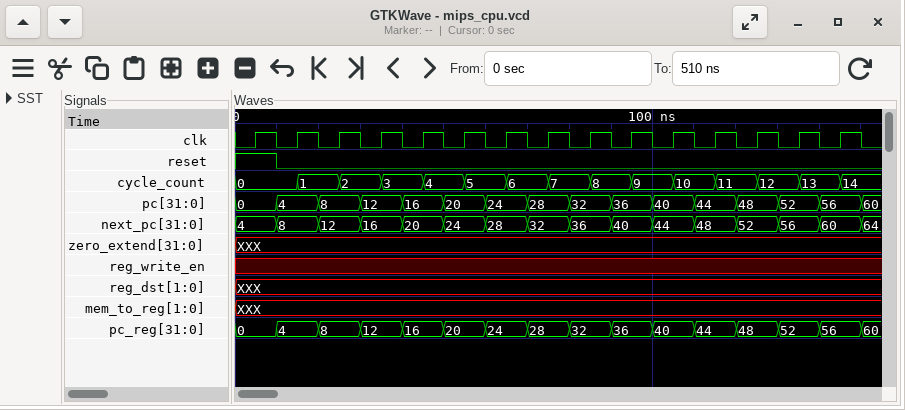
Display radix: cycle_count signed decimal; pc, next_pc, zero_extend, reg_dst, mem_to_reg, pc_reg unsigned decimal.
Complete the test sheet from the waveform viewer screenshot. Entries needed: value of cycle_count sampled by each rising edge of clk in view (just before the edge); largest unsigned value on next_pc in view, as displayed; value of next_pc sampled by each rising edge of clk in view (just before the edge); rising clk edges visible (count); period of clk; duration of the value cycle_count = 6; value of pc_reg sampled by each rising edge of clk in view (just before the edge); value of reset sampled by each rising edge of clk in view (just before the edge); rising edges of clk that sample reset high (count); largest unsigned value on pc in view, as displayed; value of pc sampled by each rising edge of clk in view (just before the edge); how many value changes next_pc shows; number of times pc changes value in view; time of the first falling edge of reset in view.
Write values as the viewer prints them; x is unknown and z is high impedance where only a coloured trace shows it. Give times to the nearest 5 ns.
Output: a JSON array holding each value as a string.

["0, 0, 1, 2, 3, 4, 5, 6, 7, 8, 9, 10, 11, 12, 13", "64", "4, 8, 12, 16, 20, 24, 28, 32, 36, 40, 44, 48, 52, 56, 60", "15", "10 ns", "10 ns", "0, 4, 8, 12, 16, 20, 24, 28, 32, 36, 40, 44, 48, 52, 56", "1 0 0 0 0 0 0 0 0 0 0 0 0 0 0", "1", "60", "0, 4, 8, 12, 16, 20, 24, 28, 32, 36, 40, 44, 48, 52, 56", "15", "15", "10 ns"]
